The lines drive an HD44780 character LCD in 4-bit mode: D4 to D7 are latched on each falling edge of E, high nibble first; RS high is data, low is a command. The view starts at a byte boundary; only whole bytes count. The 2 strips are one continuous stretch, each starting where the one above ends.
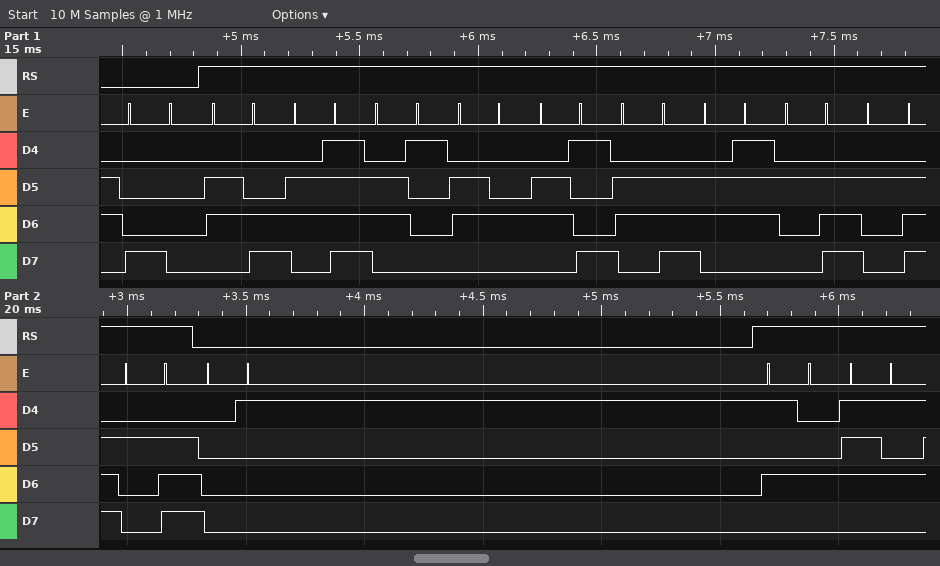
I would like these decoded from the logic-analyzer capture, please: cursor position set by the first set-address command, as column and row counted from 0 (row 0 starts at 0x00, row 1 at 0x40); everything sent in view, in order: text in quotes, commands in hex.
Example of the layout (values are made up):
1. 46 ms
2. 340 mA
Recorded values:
1. column 0, row 0
2. 0x80 "loading..." 0x01 "Tu"
